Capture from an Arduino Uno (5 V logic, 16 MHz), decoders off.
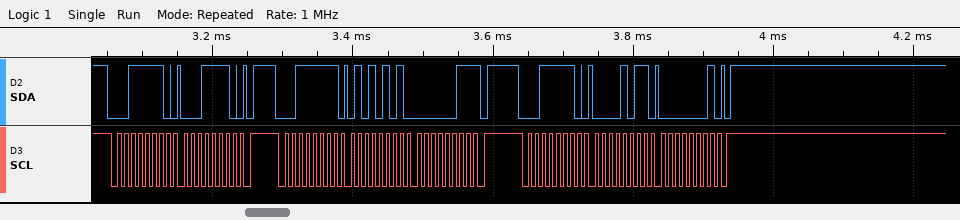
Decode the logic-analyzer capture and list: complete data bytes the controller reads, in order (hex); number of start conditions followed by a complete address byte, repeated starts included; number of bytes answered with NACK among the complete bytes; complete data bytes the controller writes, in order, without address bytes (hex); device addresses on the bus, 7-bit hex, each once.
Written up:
55 03
3
1
1E 0B 01
0x1F
